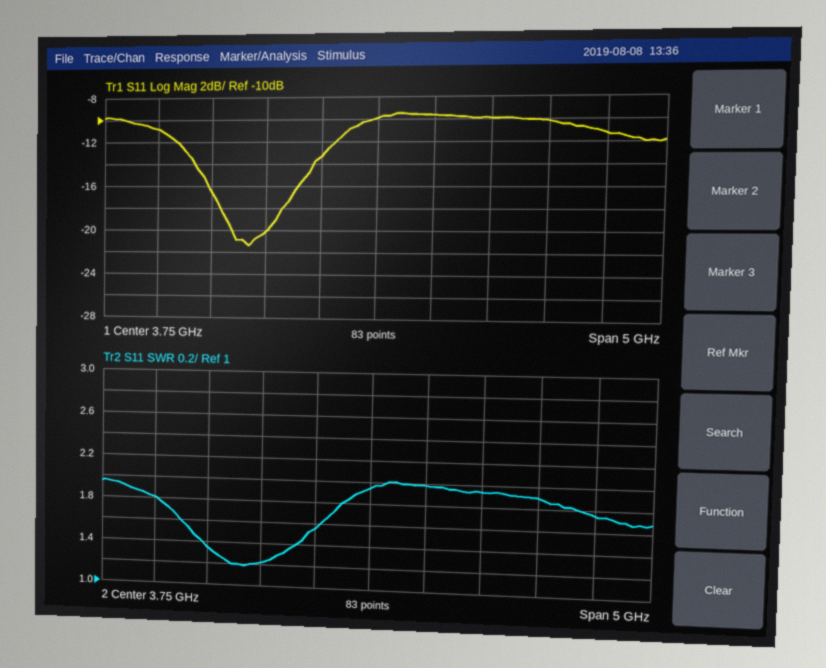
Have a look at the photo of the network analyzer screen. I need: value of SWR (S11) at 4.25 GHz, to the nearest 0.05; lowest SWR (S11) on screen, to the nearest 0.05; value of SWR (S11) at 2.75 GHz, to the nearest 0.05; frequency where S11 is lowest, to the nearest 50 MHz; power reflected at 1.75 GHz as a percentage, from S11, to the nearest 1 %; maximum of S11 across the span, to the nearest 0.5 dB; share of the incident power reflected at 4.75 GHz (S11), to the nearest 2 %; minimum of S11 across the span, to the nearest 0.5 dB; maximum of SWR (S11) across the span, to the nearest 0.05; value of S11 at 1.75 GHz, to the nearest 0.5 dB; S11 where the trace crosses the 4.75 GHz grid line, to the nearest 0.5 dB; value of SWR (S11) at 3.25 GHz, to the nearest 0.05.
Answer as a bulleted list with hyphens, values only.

- 2.00
- 1.20
- 1.20
- 2.60 GHz
- 8 %
- -9.5 dB
- 10 %
- -21.5 dB
- 2.00
- -11.0 dB
- -10.0 dB
- 1.55
